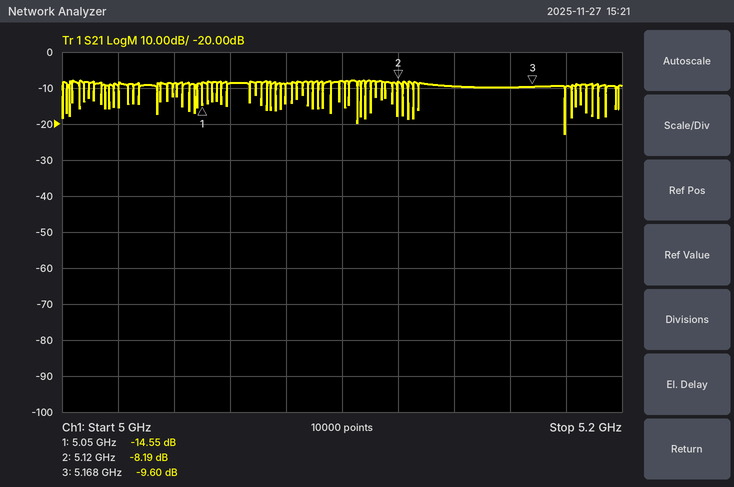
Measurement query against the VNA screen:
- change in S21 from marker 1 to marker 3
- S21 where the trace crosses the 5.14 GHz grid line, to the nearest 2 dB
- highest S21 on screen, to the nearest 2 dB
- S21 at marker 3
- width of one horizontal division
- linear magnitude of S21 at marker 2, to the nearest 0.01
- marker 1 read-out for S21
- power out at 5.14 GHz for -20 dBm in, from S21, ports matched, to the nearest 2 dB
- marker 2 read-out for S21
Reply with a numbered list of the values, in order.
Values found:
1. 4.95 dB
2. -10 dB
3. -8 dB
4. -9.60 dB
5. 20 MHz
6. 0.39
7. -14.55 dB
8. -30 dBm
9. -8.19 dB
